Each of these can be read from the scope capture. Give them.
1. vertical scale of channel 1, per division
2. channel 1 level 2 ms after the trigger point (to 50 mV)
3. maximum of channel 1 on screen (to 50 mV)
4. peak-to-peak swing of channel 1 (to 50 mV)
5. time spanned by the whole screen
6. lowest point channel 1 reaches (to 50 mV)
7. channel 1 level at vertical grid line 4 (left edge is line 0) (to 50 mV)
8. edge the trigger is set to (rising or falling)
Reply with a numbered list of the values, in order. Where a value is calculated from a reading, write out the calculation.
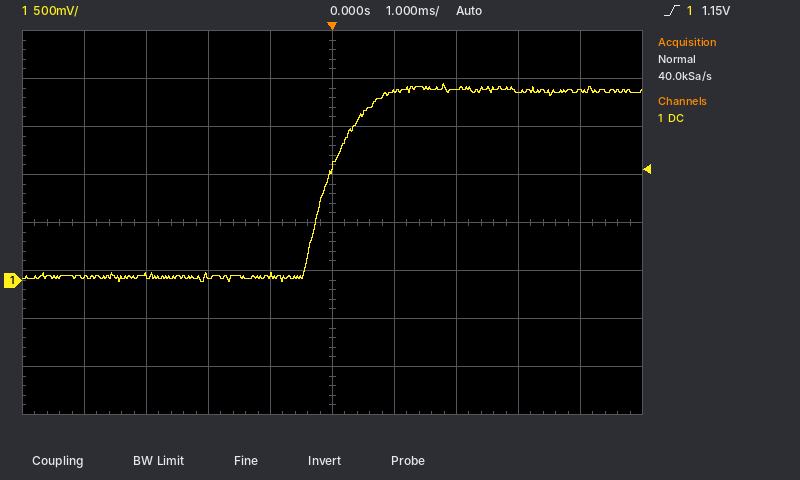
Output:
1. 500 mV
2. 2.00 V
3. 2.05 V
4. 2.05 V − (0 mV) = 2.05 V
5. 10 ms
6. 0 mV
7. 50 mV
8. rising
